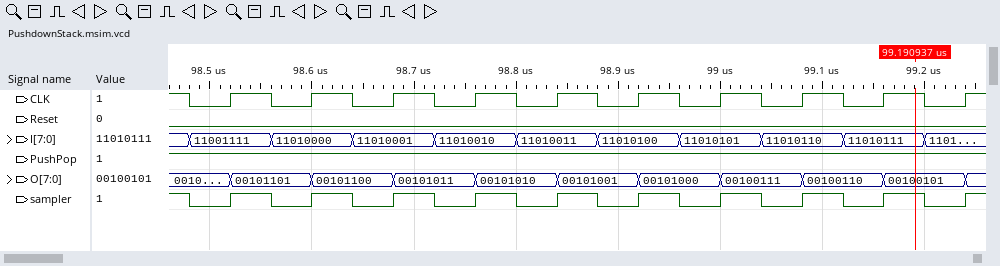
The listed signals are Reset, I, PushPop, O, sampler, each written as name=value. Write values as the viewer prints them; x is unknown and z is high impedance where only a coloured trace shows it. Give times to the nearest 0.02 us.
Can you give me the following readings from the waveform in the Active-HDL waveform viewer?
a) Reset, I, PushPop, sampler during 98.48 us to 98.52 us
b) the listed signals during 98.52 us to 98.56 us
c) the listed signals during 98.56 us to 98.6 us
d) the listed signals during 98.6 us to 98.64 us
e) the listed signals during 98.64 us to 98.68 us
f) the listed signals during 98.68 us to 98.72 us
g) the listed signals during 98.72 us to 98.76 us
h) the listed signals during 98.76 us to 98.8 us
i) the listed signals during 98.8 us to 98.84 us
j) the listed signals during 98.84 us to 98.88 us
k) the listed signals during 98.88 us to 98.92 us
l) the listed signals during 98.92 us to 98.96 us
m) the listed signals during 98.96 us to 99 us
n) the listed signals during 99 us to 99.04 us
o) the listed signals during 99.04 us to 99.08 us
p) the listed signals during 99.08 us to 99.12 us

Reset=0, I=11001111, PushPop=1, sampler=0
Reset=0, I=11001111, PushPop=1, O=00101101, sampler=1
Reset=0, I=11010000, PushPop=1, O=00101101, sampler=0
Reset=0, I=11010000, PushPop=1, O=00101100, sampler=1
Reset=0, I=11010001, PushPop=1, O=00101100, sampler=0
Reset=0, I=11010001, PushPop=1, O=00101011, sampler=1
Reset=0, I=11010010, PushPop=1, O=00101011, sampler=0
Reset=0, I=11010010, PushPop=1, O=00101010, sampler=1
Reset=0, I=11010011, PushPop=1, O=00101010, sampler=0
Reset=0, I=11010011, PushPop=1, O=00101001, sampler=1
Reset=0, I=11010100, PushPop=1, O=00101001, sampler=0
Reset=0, I=11010100, PushPop=1, O=00101000, sampler=1
Reset=0, I=11010101, PushPop=1, O=00101000, sampler=0
Reset=0, I=11010101, PushPop=1, O=00100111, sampler=1
Reset=0, I=11010110, PushPop=1, O=00100111, sampler=0
Reset=0, I=11010110, PushPop=1, O=00100110, sampler=1
